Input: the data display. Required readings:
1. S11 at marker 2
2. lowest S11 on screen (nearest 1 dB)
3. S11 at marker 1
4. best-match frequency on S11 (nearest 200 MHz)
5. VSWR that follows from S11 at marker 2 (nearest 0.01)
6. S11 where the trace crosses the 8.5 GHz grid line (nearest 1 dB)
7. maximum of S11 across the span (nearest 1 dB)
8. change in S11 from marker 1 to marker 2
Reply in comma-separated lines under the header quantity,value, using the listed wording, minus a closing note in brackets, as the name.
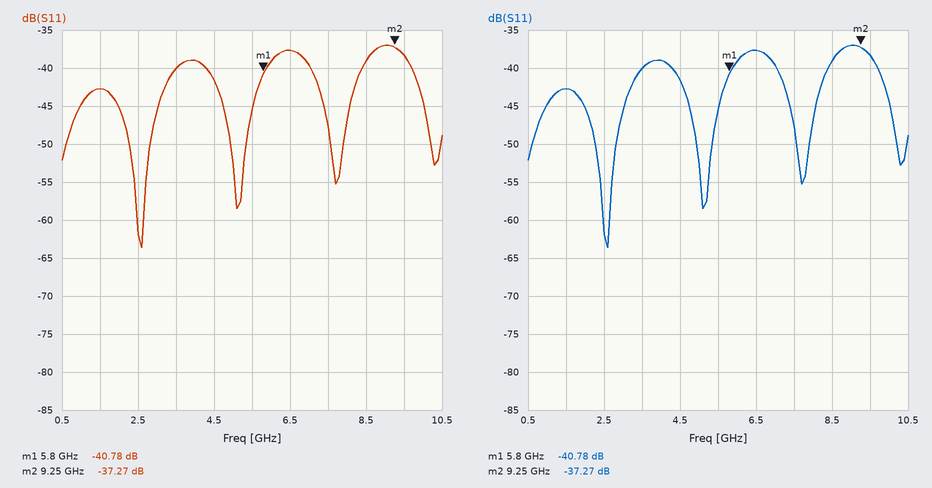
quantity,value
S11 at marker 2,-37.27 dB
lowest S11 on screen,-64 dB
S11 at marker 1,-40.78 dB
best-match frequency on S11,2.6 GHz
VSWR that follows from S11 at marker 2,1.03
S11 where the trace crosses the 8.5 GHz grid line,-39 dB
maximum of S11 across the span,-37 dB
change in S11 from marker 1 to marker 2,3.51 dB
